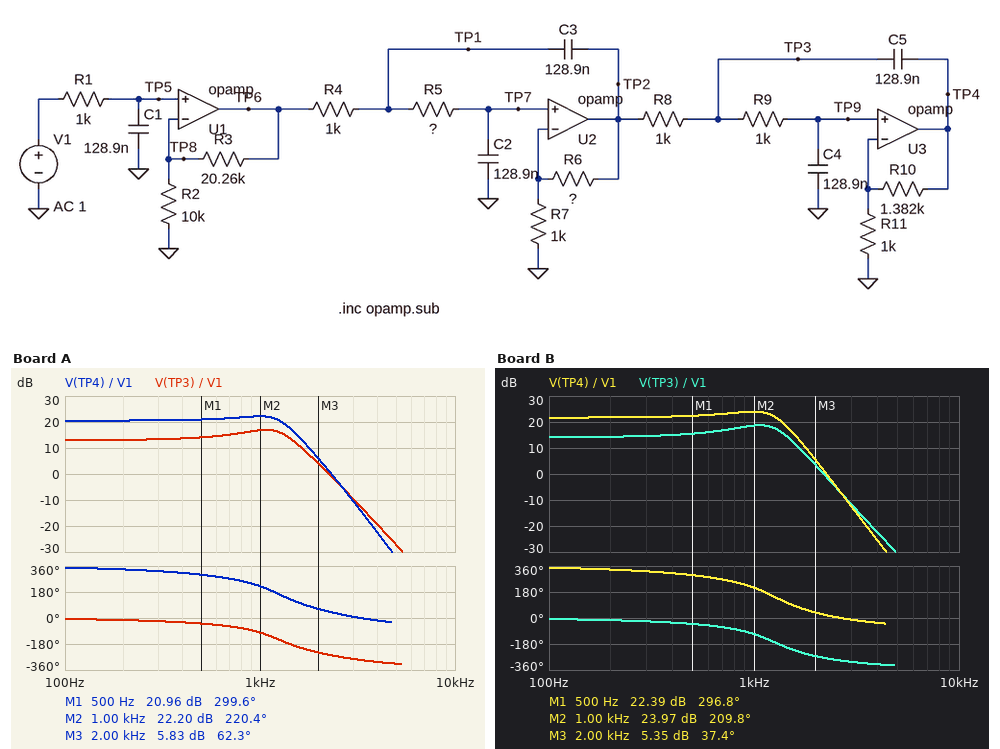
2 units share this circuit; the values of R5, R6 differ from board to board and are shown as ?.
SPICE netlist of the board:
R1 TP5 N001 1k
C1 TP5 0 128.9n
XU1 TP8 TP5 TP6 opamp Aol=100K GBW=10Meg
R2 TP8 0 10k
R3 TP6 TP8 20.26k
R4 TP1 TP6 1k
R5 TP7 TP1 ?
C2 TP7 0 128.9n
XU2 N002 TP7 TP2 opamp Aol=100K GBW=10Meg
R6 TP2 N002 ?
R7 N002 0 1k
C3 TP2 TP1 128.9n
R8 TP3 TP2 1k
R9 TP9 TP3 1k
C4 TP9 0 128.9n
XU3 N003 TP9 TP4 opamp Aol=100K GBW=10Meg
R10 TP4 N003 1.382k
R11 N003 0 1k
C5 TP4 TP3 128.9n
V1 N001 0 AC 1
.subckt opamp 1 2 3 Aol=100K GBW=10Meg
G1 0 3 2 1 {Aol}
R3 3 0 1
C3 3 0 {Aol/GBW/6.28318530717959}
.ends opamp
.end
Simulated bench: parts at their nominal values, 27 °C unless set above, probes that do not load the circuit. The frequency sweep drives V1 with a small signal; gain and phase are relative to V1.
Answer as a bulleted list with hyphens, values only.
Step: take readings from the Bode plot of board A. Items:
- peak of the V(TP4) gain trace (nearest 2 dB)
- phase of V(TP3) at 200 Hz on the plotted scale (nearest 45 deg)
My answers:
- 22 dB
- 0 deg
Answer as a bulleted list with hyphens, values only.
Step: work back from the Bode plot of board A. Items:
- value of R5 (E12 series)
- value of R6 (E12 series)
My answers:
- 390 Ω
- 470 Ω
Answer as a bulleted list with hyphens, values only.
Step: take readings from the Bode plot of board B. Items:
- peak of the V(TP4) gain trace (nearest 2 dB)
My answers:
- 24 dB
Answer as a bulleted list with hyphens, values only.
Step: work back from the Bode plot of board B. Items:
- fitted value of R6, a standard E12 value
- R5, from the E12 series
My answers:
- 680 Ω
- 680 Ω
